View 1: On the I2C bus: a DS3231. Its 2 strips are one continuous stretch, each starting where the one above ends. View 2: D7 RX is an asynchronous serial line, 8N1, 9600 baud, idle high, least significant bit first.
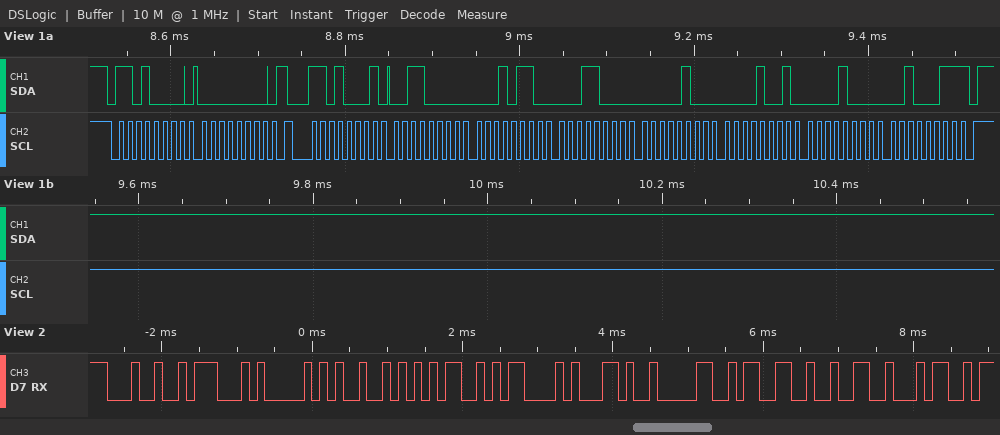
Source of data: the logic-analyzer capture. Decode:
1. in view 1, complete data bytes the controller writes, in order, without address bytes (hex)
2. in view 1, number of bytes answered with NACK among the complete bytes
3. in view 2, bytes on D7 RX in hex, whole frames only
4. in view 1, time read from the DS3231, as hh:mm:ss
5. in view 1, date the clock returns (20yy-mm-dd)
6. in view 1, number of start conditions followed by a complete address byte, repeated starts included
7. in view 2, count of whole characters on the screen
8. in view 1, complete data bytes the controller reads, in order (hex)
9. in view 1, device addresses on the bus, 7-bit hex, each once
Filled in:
00
1
24 47 50 52 4D 43 2C 30 33 32 34
18:16:30
2023-08-09
2
11
30 16 18 04 09 08 23
0x68
